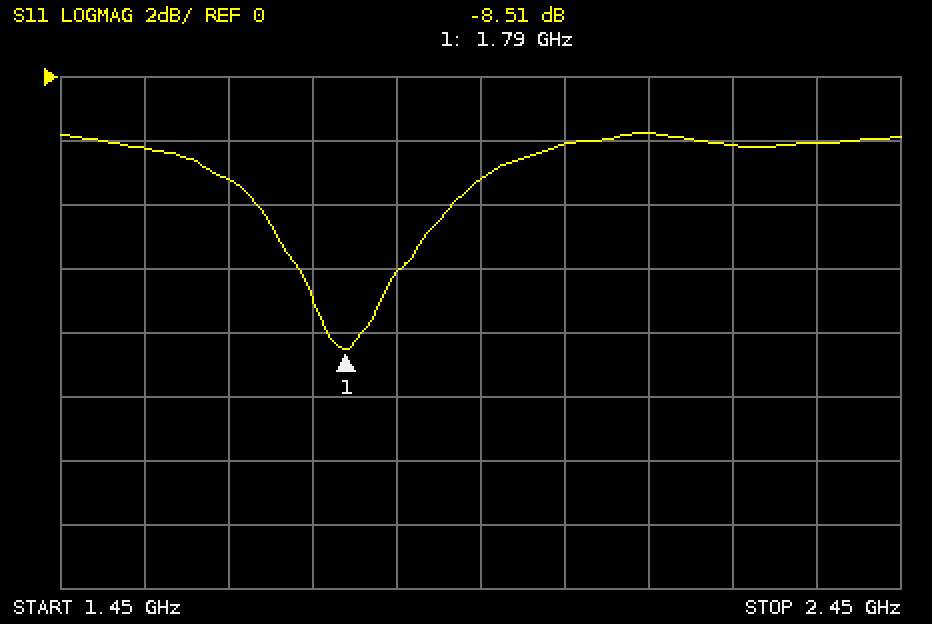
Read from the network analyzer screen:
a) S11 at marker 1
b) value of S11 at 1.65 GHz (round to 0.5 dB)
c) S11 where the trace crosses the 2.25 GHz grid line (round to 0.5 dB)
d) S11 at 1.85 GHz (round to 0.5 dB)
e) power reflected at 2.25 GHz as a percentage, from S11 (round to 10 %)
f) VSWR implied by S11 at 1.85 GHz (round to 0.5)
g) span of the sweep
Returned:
-8.51 dB
-3.0 dB
-2.0 dB
-6.0 dB
60 %
3.0
1 GHz
